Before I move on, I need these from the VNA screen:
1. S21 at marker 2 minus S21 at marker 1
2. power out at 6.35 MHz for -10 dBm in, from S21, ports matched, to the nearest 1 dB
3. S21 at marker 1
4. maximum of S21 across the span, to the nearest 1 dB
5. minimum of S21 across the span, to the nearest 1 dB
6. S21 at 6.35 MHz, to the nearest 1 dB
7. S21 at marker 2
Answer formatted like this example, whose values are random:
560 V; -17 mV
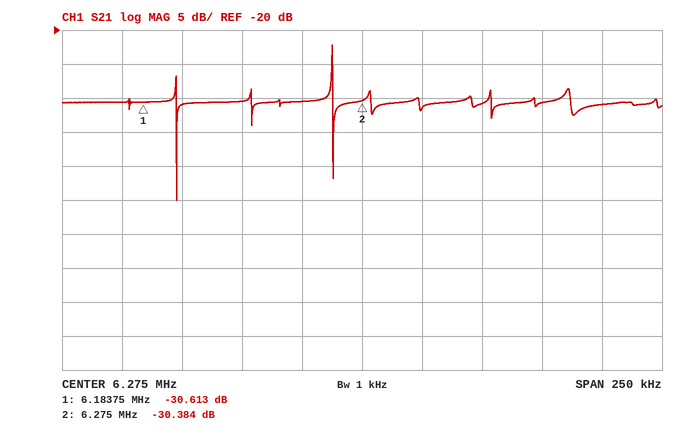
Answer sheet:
0.229 dB; -41 dBm; -30.613 dB; -22 dB; -45 dB; -31 dB; -30.384 dB
